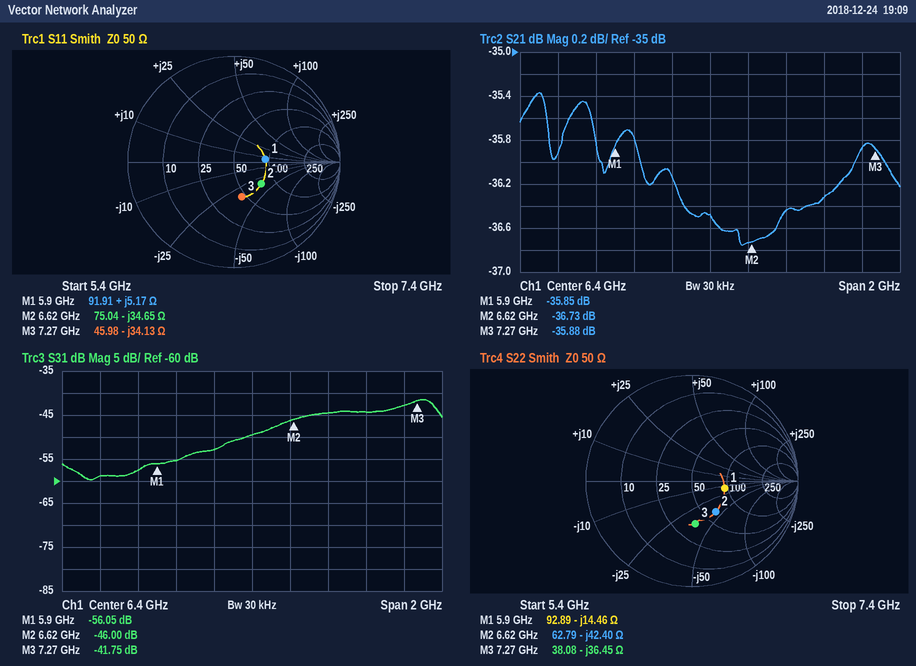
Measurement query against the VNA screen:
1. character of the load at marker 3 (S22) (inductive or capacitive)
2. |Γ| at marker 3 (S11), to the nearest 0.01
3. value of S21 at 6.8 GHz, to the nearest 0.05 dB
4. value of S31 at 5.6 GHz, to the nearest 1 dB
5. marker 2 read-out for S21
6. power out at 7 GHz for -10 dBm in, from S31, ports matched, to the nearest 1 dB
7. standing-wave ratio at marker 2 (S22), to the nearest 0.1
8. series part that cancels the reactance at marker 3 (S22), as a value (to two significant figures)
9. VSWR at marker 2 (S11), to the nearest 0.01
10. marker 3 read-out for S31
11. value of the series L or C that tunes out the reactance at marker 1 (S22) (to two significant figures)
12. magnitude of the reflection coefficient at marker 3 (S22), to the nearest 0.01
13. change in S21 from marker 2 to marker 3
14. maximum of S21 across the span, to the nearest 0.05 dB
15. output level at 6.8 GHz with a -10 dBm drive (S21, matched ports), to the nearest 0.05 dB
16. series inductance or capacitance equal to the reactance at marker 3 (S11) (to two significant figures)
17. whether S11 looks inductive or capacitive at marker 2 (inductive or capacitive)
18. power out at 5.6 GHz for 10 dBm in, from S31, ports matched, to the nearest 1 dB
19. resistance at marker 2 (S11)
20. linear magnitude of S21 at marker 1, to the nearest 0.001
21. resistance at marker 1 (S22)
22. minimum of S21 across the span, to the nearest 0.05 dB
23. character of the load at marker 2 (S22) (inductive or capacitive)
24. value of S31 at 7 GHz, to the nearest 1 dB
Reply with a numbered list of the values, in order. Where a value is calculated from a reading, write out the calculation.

1. capacitive
2. 0.34
3. -36.45 dB
4. -59 dB
5. -36.73 dB
6. -10 dBm + (-44 dB) = -54 dBm
7. 2.2
8. L = 36.45 Ω/(2π × 7.27 GHz) ≈ 798 pH, so 800 pH to two significant figures
9. 1.98
10. -41.75 dB
11. L = 14.46 Ω/(2π × 5.9 GHz) ≈ 390 pH
12. 0.40
13. -35.88 − (-36.73) = 0.85 dB
14. -35.35 dB
15. -10 dBm + (-36.45 dB) = -46.45 dBm
16. C = 1/(2π × 7.27 GHz × 34.13 Ω) ≈ 641 fF, so 640 fF to two significant figures
17. capacitive
18. 10 dBm + (-59 dB) = -49 dBm
19. 75.04 Ω
20. 10^(-35.85/20) ≈ 0.016
21. 92.89 Ω
22. -36.75 dB
23. capacitive
24. -44 dB
